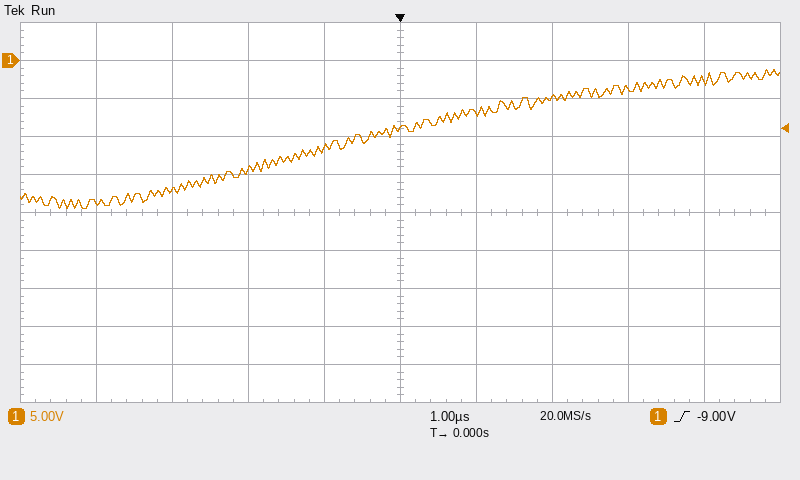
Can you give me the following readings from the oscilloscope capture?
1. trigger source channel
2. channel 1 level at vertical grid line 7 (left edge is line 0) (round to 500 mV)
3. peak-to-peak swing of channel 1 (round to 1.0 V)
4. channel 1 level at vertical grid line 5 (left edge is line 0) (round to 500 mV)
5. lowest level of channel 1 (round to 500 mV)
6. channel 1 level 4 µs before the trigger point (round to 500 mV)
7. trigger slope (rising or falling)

channel 1
-5.0 V
18.0 V
-9.0 V
-19.5 V
-18.5 V
rising
